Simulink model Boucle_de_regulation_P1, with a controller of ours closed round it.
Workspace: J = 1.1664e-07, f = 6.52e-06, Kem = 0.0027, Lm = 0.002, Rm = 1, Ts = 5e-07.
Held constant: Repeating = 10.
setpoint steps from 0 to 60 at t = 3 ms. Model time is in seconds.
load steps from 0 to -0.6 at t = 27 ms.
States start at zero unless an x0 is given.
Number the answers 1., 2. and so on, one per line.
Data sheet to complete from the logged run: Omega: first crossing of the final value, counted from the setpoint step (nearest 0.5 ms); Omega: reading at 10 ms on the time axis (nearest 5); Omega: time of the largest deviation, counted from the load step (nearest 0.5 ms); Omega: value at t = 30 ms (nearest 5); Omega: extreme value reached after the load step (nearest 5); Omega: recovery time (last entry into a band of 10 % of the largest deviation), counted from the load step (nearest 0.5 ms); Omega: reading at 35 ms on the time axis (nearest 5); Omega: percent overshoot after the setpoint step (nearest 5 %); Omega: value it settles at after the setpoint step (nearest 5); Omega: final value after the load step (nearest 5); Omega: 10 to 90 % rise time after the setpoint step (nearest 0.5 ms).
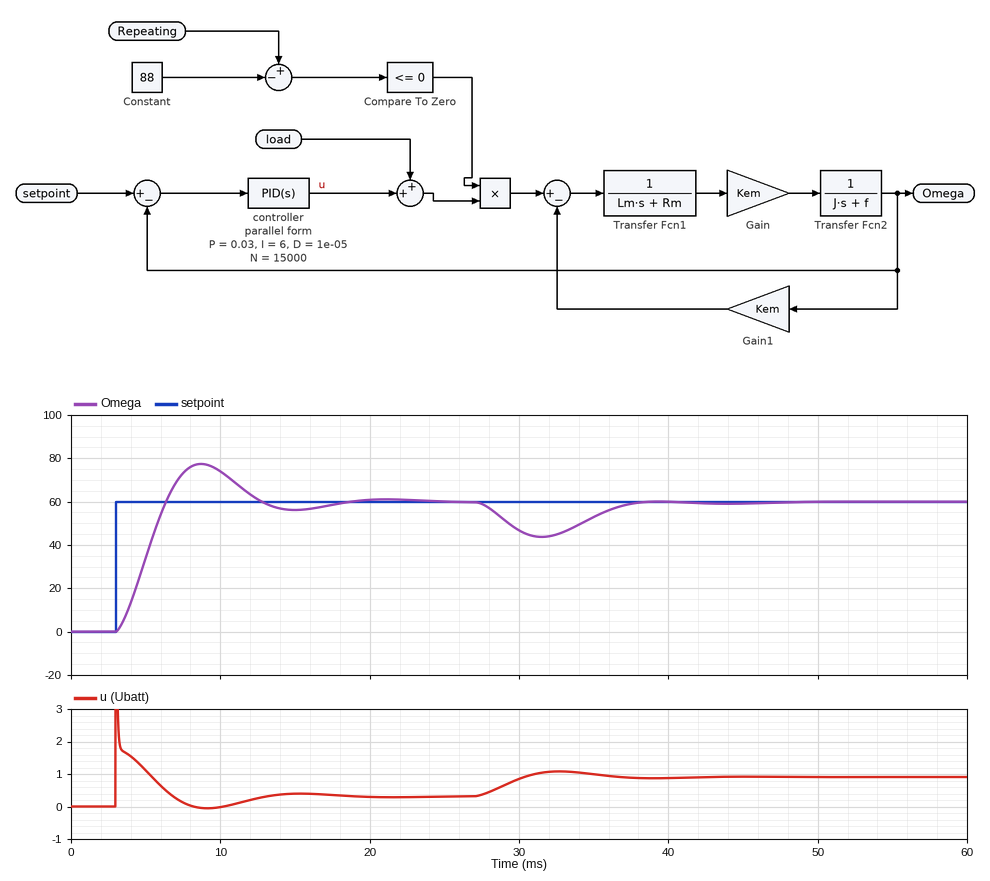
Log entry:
1. 3.5 ms
2. 75
3. 4.5 ms
4. 45
5. 45
6. 10.0 ms
7. 55
8. 30 %
9. 60
10. 60
11. 2.5 ms
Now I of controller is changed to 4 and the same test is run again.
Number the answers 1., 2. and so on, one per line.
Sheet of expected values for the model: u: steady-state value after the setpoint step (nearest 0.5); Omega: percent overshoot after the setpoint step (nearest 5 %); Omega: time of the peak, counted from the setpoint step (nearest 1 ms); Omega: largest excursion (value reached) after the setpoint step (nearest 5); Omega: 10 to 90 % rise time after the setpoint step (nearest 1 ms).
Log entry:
1. 0.5
2. 20 %
3. 6 ms
4. 70
5. 3 ms
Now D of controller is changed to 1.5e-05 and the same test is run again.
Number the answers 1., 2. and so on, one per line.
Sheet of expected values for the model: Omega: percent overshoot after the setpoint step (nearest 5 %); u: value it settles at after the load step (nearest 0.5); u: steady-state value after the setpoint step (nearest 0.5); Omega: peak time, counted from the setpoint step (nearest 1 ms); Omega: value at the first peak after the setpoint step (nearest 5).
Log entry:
1. 25 %
2. 1.0
3. 0.5
4. 6 ms
5. 75
